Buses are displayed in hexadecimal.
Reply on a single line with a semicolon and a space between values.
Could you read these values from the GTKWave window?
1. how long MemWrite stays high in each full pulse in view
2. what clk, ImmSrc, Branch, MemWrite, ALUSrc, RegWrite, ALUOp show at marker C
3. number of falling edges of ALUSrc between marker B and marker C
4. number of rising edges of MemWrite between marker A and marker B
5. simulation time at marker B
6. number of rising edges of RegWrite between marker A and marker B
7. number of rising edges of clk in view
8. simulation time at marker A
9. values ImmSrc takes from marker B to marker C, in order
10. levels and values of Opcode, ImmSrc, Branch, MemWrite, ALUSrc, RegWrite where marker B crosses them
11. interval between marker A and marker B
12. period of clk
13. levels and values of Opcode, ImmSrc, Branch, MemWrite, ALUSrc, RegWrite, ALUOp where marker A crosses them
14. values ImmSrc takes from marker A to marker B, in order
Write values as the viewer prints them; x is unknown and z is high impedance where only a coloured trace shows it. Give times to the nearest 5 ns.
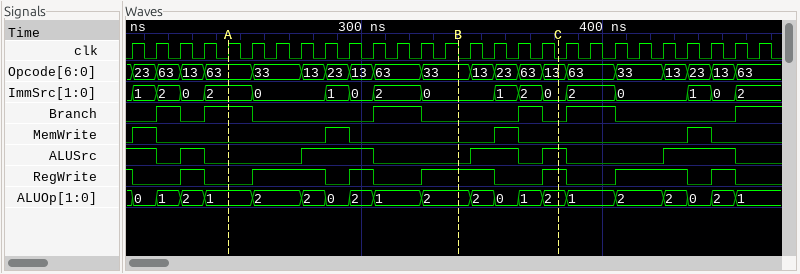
10 ns, 10 ns, 10 ns, 10 ns; clk=0, ImmSrc=0, Branch=0, MemWrite=0, ALUSrc=1, RegWrite=1, ALUOp=2; 1; 1; 340 ns; 3; 27; 245 ns; 0, 1, 2, 0; Opcode=33, ImmSrc=0, Branch=0, MemWrite=0, ALUSrc=0, RegWrite=1; 95 ns; 10 ns; Opcode=63, ImmSrc=2, Branch=1, MemWrite=0, ALUSrc=0, RegWrite=0, ALUOp=1; 2, 0, 1, 0, 2, 0
